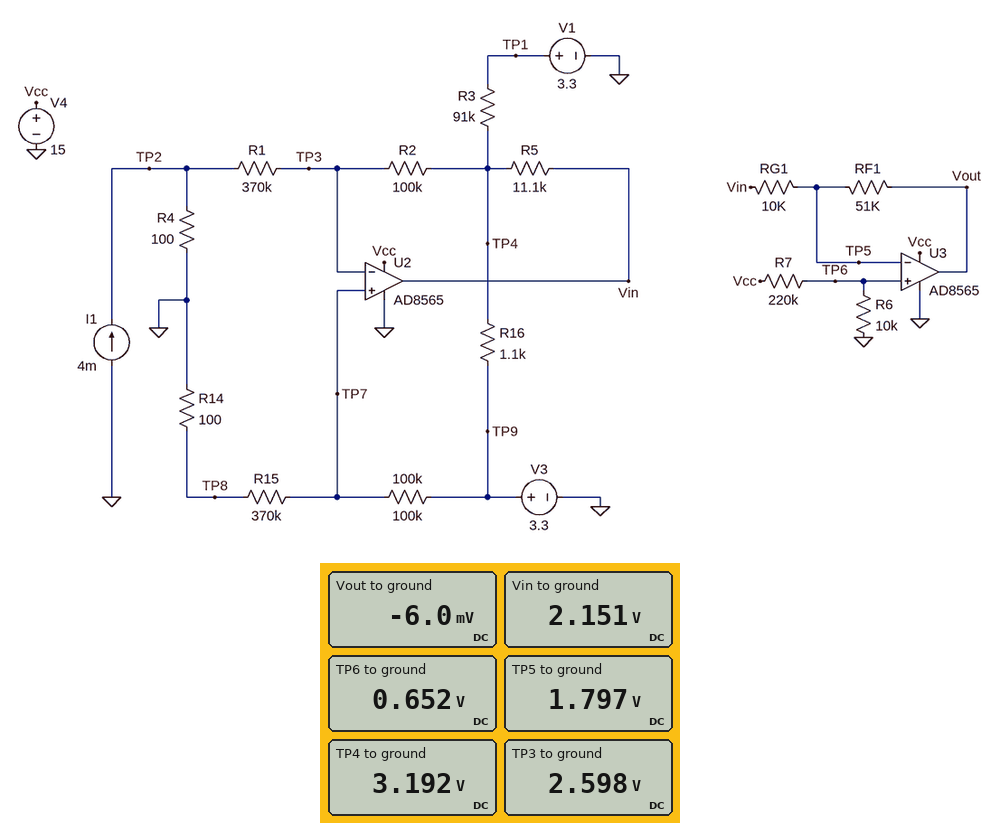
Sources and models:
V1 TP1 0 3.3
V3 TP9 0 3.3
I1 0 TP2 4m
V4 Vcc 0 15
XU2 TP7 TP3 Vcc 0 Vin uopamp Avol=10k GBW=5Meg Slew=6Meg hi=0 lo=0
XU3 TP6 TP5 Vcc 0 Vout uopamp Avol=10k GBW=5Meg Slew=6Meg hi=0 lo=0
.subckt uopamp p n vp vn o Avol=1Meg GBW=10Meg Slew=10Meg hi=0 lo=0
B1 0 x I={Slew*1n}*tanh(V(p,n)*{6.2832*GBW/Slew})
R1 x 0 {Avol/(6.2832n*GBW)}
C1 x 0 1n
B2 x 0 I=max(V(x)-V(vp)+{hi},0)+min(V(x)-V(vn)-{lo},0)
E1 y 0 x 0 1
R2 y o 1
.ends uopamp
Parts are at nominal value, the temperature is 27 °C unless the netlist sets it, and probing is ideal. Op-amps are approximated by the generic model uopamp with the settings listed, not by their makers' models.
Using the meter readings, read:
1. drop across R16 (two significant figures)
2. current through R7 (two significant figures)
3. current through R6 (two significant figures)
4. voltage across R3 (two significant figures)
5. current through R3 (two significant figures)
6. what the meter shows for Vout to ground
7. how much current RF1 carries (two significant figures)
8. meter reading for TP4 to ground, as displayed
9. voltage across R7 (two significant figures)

110 mV
65 µA
65 µA
110 mV
1.2 µA
-6.0 mV
35 µA
3.192 V
14 V
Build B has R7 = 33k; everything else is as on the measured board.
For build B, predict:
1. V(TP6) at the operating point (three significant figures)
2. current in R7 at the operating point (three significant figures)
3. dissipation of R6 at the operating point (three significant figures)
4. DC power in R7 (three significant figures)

3.49 V
349 µA
1.22 mW
4.02 mW
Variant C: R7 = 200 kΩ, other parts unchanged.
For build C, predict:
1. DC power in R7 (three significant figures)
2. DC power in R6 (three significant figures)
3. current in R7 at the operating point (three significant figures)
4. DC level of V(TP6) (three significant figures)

1.02 mW
51.0 µW
71.4 µA
714 mV
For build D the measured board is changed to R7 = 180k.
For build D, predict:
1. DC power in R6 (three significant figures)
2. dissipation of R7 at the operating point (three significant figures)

62.3 µW
1.12 mW
